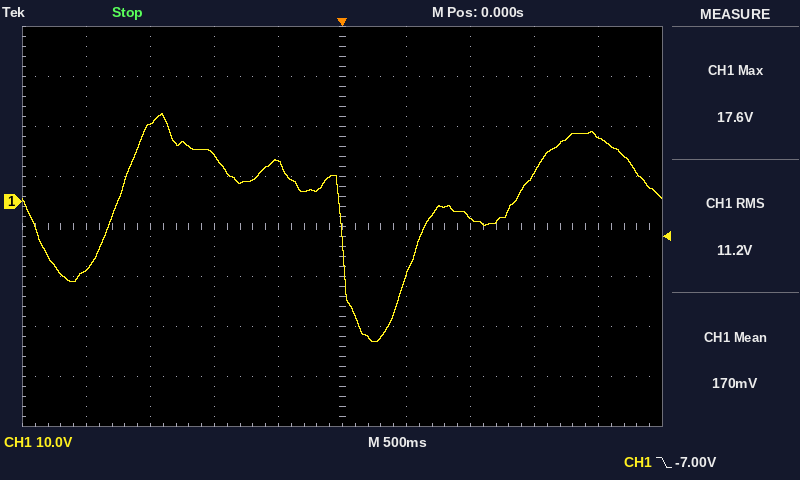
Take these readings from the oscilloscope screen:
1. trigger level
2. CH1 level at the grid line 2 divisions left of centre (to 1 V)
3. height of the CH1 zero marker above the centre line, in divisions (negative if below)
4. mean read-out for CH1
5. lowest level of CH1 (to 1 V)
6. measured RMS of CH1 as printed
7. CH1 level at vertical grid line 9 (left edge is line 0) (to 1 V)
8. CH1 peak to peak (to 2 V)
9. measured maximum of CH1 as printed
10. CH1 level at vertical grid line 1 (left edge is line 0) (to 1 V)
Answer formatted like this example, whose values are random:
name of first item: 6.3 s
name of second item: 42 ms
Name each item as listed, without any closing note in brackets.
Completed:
trigger level: -7.00 V
CH1 level at the grid line 2 divisions left of centre: 9 V
height of the CH1 zero marker above the centre line, in divisions: +0.5 div
mean read-out for CH1: 170 mV
lowest level of CH1: -28 V
measured RMS of CH1 as printed: 11.2 V
CH1 level at vertical grid line 9 (left edge is line 0): 13 V
CH1 peak to peak: 46 V
measured maximum of CH1 as printed: 17.6 V
CH1 level at vertical grid line 1 (left edge is line 0): -14 V
